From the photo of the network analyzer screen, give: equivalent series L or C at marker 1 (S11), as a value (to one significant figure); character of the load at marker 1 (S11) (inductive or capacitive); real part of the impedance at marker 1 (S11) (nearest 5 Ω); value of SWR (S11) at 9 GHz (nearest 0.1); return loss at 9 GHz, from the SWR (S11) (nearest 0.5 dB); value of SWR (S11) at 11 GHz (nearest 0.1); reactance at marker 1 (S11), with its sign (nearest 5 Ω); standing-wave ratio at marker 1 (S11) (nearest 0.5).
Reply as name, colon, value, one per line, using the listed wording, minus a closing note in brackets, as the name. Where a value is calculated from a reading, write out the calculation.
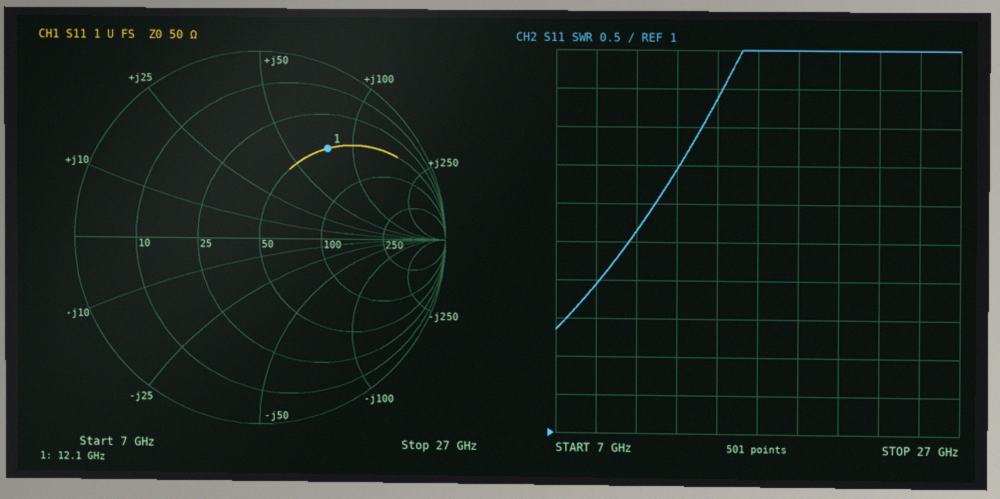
equivalent series L or C at marker 1 (S11), as a value: L = 75 Ω/(2π × 12.1 GHz) ≈ 1.0 nH
character of the load at marker 1 (S11): inductive
real part of the impedance at marker 1 (S11): 50 Ω
value of SWR (S11) at 9 GHz: 2.9
return loss at 9 GHz, from the SWR (S11): −20 log10((2.9 − 1)/(2.9 + 1)) ≈ 6.25 dB, so 6.0 dB to the nearest 0.5 dB
value of SWR (S11) at 11 GHz: 3.6
reactance at marker 1 (S11), with its sign: +75 Ω
standing-wave ratio at marker 1 (S11): 4.0
